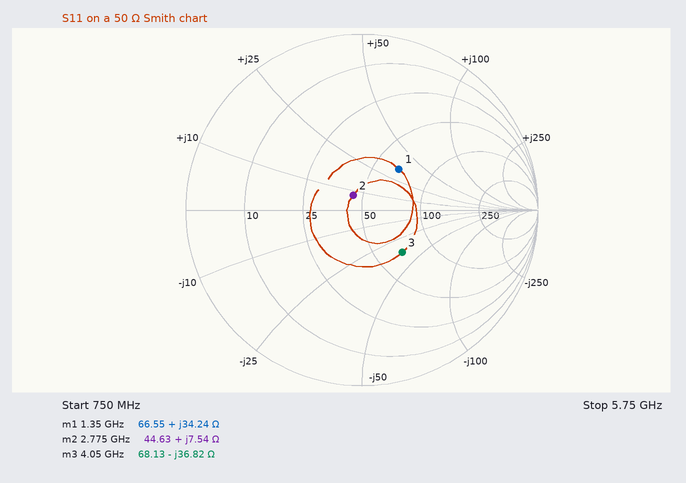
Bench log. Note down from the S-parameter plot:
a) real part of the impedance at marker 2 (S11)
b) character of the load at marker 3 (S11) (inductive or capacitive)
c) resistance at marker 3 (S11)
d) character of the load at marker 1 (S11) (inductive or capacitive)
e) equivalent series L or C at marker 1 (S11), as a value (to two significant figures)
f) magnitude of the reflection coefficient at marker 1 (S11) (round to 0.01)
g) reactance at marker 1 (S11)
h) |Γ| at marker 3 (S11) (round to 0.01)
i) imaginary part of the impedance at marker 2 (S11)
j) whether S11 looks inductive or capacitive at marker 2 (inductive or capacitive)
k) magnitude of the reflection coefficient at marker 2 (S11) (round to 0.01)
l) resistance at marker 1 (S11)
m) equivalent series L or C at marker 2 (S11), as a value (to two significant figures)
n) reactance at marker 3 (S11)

44.63 Ω
capacitive
68.13 Ω
inductive
4.0 nH
0.31
+34.24 Ω
0.33
+7.54 Ω
inductive
0.10
66.55 Ω
430 pH
-36.82 Ω
